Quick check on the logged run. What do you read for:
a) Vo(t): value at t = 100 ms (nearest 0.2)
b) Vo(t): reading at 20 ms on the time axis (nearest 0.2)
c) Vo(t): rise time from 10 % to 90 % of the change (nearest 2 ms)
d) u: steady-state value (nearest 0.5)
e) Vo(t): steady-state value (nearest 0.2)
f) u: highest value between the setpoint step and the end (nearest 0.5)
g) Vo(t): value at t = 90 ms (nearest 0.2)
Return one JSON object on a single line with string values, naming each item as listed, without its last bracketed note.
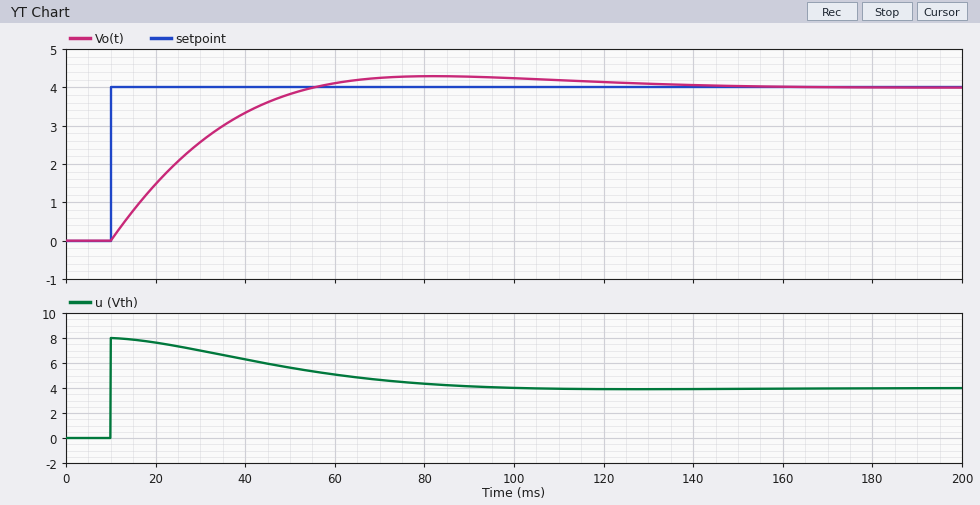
{"Vo(t): value at t = 100 ms": "4.2", "Vo(t): reading at 20 ms on the time axis": "1.4", "Vo(t): rise time from 10 % to 90 % of the change": "32 ms", "u: steady-state value": "4.0", "Vo(t): steady-state value": "4.0", "u: highest value between the setpoint step and the end": "8.0", "Vo(t): value at t = 90 ms": "4.2"}
